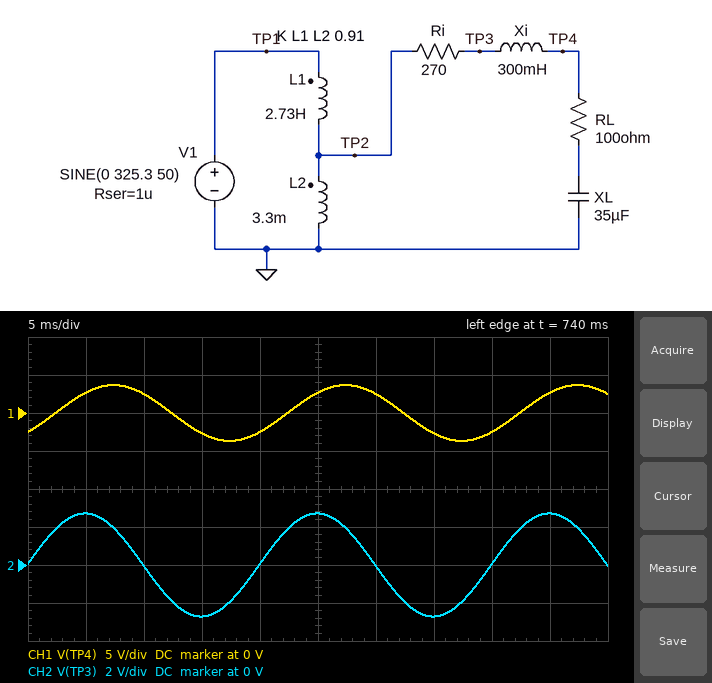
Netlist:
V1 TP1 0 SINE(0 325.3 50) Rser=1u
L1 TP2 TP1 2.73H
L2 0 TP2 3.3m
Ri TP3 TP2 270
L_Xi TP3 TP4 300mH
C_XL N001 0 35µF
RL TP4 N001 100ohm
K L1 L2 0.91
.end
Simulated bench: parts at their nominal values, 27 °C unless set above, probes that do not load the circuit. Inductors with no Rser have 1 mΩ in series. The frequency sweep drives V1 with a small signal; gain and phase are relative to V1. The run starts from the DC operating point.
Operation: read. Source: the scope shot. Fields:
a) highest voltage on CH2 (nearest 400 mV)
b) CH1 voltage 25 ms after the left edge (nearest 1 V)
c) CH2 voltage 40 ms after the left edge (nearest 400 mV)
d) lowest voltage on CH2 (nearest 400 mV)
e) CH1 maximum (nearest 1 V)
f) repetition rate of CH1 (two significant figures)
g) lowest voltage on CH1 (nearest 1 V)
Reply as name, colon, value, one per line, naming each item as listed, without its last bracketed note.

highest voltage on CH2: 2.8 V
CH1 voltage 25 ms after the left edge: 3 V
CH2 voltage 40 ms after the left edge: 0 V
lowest voltage on CH2: -2.8 V
CH1 maximum: 4 V
repetition rate of CH1: 50 Hz
lowest voltage on CH1: -4 V
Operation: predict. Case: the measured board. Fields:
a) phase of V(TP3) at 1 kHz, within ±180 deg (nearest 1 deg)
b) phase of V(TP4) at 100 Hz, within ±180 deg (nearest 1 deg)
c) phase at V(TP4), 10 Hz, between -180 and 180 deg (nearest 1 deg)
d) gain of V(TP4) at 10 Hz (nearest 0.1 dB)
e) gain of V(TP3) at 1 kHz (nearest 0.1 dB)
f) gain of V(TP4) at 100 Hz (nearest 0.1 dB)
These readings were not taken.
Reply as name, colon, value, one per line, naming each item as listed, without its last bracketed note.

phase of V(TP3) at 1 kHz, within ±180 deg: 8 deg
phase of V(TP4) at 100 Hz, within ±180 deg: -46 deg
phase at V(TP4), 10 Hz, between -180 and 180 deg: -28 deg
gain of V(TP4) at 10 Hz: -32.0 dB
gain of V(TP3) at 1 kHz: -30.4 dB
gain of V(TP4) at 100 Hz: -41.4 dB
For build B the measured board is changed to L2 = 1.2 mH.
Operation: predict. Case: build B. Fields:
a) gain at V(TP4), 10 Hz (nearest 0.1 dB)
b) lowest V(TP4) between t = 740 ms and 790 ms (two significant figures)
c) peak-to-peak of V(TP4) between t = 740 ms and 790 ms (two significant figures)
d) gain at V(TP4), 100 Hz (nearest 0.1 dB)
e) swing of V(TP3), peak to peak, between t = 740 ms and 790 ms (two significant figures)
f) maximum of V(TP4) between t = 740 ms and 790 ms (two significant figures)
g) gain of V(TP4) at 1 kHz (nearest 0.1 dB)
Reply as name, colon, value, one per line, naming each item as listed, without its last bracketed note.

gain at V(TP4), 10 Hz: -36.3 dB
lowest V(TP4) between t = 740 ms and 790 ms: -2.2 V
peak-to-peak of V(TP4) between t = 740 ms and 790 ms: 4.5 V
gain at V(TP4), 100 Hz: -45.7 dB
swing of V(TP3), peak to peak, between t = 740 ms and 790 ms: 3.3 V
maximum of V(TP4) between t = 740 ms and 790 ms: 2.2 V
gain of V(TP4) at 1 kHz: -60.2 dB
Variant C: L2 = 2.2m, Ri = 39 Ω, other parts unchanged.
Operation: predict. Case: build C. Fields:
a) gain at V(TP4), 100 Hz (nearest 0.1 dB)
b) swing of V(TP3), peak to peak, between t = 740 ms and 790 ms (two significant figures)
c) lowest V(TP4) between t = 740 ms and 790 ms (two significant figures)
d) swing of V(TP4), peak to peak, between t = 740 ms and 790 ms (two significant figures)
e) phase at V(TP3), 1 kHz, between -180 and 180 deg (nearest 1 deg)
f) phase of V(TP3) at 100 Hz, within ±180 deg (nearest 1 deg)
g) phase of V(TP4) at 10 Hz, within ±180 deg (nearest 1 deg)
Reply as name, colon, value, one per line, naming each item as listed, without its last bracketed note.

gain at V(TP4), 100 Hz: -37.1 dB
swing of V(TP3), peak to peak, between t = 740 ms and 790 ms: 12 V
lowest V(TP4) between t = 740 ms and 790 ms: -8.0 V
swing of V(TP4), peak to peak, between t = 740 ms and 790 ms: 16 V
phase at V(TP3), 1 kHz, between -180 and 180 deg: 1 deg
phase of V(TP3) at 100 Hz, within ±180 deg: 9 deg
phase of V(TP4) at 10 Hz, within ±180 deg: -5 deg
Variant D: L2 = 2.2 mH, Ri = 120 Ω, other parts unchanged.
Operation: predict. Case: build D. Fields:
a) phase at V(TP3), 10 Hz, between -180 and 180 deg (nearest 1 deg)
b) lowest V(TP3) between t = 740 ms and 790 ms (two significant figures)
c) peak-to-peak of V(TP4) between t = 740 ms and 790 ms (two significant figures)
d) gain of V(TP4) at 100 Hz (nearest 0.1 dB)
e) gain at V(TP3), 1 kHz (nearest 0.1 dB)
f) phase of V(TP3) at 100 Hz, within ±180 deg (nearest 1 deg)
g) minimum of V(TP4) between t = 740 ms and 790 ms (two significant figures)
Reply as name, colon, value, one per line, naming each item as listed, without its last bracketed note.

phase at V(TP3), 10 Hz, between -180 and 180 deg: -14 deg
lowest V(TP3) between t = 740 ms and 790 ms: -3.7 V
peak-to-peak of V(TP4) between t = 740 ms and 790 ms: 10 V
gain of V(TP4) at 100 Hz: -39.5 dB
gain at V(TP3), 1 kHz: -32.0 dB
phase of V(TP3) at 100 Hz, within ±180 deg: 22 deg
minimum of V(TP4) between t = 740 ms and 790 ms: -5.1 V
